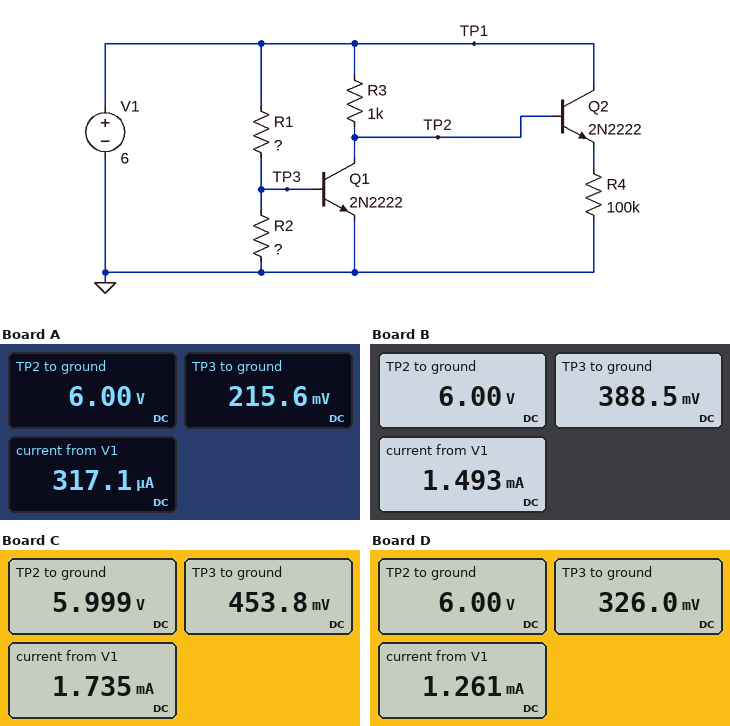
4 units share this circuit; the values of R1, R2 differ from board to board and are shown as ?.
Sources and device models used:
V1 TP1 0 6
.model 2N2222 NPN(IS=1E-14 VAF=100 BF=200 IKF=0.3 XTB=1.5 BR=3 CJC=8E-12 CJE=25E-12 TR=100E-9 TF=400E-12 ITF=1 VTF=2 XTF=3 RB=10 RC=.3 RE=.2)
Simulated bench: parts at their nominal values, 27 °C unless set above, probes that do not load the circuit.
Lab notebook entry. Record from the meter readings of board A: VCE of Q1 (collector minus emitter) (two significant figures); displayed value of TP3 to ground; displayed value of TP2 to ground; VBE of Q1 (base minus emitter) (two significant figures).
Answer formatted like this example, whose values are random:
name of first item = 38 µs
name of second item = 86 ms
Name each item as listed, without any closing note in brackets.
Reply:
VCE of Q1 (collector minus emitter) = 6.0 V
displayed value of TP3 to ground = 215.6 mV
displayed value of TP2 to ground = 6.00 V
VBE of Q1 (base minus emitter) = 220 mV
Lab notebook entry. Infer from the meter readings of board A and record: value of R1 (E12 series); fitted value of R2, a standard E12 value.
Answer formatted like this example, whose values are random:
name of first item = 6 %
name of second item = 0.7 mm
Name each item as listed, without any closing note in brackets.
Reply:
value of R1 = 22 kΩ
fitted value of R2, a standard E12 value = 820 Ω
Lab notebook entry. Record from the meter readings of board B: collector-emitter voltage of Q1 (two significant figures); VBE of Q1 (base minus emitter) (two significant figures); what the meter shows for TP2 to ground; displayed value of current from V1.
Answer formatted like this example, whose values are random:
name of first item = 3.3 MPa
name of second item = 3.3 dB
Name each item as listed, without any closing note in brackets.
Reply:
collector-emitter voltage of Q1 = 6.0 V
VBE of Q1 (base minus emitter) = 390 mV
what the meter shows for TP2 to ground = 6.00 V
displayed value of current from V1 = 1.493 mA
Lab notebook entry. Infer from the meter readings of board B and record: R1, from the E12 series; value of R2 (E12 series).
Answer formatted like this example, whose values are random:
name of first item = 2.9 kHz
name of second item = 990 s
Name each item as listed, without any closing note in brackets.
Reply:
R1, from the E12 series = 3.9 kΩ
value of R2 = 270 Ω
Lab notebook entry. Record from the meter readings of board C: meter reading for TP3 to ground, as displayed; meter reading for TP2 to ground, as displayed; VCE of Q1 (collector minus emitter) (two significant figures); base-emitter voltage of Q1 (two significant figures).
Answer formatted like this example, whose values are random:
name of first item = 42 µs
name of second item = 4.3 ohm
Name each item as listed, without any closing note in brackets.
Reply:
meter reading for TP3 to ground, as displayed = 453.8 mV
meter reading for TP2 to ground, as displayed = 5.999 V
VCE of Q1 (collector minus emitter) = 6.0 V
base-emitter voltage of Q1 = 450 mV
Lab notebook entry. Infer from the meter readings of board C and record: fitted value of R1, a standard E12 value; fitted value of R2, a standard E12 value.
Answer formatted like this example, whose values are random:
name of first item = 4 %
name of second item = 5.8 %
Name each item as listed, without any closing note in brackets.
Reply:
fitted value of R1, a standard E12 value = 3.3 kΩ
fitted value of R2, a standard E12 value = 270 Ω
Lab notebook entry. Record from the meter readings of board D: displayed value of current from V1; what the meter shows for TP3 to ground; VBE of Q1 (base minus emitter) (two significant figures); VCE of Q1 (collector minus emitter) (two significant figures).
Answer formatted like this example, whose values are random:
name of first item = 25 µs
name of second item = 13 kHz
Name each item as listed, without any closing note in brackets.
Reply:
displayed value of current from V1 = 1.261 mA
what the meter shows for TP3 to ground = 326.0 mV
VBE of Q1 (base minus emitter) = 330 mV
VCE of Q1 (collector minus emitter) = 6.0 V
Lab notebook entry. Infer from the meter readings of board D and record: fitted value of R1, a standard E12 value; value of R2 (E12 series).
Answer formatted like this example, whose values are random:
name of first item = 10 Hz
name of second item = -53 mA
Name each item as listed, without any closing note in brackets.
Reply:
fitted value of R1, a standard E12 value = 4.7 kΩ
value of R2 = 270 Ω
